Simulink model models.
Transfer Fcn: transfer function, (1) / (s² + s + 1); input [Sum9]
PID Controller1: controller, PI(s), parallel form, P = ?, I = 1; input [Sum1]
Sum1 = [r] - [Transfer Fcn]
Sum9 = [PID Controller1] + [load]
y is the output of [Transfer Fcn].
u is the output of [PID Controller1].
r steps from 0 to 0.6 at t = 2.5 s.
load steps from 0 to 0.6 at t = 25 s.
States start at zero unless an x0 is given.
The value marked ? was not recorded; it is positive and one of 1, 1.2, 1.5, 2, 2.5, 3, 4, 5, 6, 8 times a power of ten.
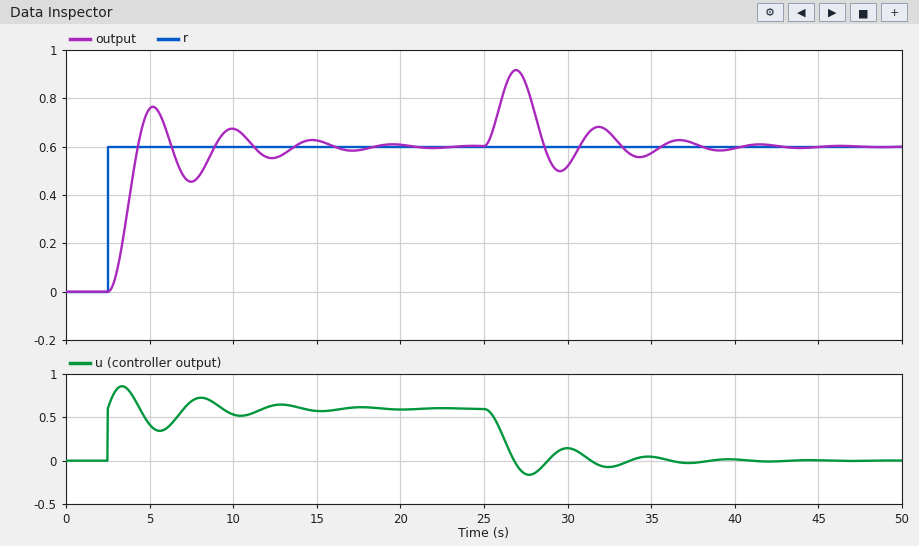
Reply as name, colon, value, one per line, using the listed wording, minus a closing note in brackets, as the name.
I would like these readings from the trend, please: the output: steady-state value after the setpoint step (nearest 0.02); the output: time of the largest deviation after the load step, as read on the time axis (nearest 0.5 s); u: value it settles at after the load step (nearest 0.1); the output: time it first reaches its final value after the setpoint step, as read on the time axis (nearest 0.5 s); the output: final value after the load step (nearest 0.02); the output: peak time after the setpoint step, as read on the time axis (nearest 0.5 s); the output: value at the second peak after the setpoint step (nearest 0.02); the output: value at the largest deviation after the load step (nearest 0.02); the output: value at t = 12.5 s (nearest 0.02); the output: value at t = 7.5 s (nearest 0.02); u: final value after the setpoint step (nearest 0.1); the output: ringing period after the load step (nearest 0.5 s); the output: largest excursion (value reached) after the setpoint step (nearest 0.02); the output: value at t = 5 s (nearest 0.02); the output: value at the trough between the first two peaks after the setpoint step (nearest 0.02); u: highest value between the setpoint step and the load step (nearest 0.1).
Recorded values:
the output: steady-state value after the setpoint step: 0.60
the output: time of the largest deviation after the load step, as read on the time axis: 27.0 s
u: value it settles at after the load step: 0.0
the output: time it first reaches its final value after the setpoint step, as read on the time axis: 4.5 s
the output: final value after the load step: 0.60
the output: peak time after the setpoint step, as read on the time axis: 5.0 s
the output: value at the second peak after the setpoint step: 0.68
the output: value at the largest deviation after the load step: 0.92
the output: value at t = 12.5 s: 0.56
the output: value at t = 7.5 s: 0.46
u: final value after the setpoint step: 0.6
the output: ringing period after the load step: 5.0 s
the output: largest excursion (value reached) after the setpoint step: 0.76
the output: value at t = 5 s: 0.76
the output: value at the trough between the first two peaks after the setpoint step: 0.46
u: highest value between the setpoint step and the load step: 0.9
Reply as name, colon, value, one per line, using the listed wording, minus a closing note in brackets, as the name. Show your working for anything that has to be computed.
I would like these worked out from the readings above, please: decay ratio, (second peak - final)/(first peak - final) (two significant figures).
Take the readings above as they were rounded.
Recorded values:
decay ratio, (second peak - final)/(first peak - final): (0.68 - 0.6) / (0.76 - 0.6) = 0.50
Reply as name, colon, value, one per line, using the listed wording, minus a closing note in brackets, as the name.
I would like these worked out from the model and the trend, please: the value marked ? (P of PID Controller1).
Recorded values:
the value marked ?: 1
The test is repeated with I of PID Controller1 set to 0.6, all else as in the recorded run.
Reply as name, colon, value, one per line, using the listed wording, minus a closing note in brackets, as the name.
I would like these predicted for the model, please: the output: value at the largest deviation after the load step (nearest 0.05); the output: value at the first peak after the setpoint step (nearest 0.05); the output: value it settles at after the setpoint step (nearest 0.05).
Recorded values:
the output: value at the largest deviation after the load step: 0.95
the output: value at the first peak after the setpoint step: 0.65
the output: value it settles at after the setpoint step: 0.60
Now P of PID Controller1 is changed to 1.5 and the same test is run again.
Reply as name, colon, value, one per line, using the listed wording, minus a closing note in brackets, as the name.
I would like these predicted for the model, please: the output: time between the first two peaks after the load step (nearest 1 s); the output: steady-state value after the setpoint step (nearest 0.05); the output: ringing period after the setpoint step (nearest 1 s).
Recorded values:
the output: time between the first two peaks after the load step: 4 s
the output: steady-state value after the setpoint step: 0.60
the output: ringing period after the setpoint step: 4 s
